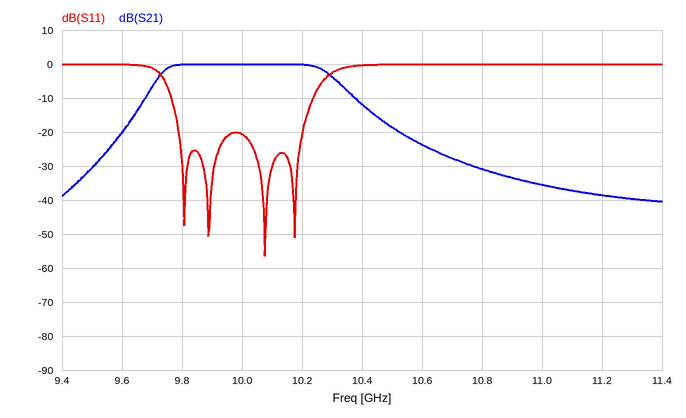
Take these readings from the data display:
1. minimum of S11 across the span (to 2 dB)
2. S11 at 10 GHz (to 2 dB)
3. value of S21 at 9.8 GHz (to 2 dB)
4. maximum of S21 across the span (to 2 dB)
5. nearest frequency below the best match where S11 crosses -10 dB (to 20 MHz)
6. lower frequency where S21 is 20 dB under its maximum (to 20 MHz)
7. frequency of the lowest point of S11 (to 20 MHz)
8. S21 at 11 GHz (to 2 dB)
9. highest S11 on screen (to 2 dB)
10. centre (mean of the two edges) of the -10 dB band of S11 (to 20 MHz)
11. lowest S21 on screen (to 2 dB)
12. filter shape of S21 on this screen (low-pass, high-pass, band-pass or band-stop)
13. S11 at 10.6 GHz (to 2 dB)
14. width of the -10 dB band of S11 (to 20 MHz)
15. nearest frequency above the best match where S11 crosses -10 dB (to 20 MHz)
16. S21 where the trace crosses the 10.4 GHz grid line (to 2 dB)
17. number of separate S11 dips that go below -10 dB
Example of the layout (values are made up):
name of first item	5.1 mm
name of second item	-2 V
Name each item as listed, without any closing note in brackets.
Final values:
minimum of S11 across the span	-56 dB
S11 at 10 GHz	-20 dB
value of S21 at 9.8 GHz	0 dB
maximum of S21 across the span	0 dB
nearest frequency below the best match where S11 crosses -10 dB	9.76 GHz
lower frequency where S21 is 20 dB under its maximum	9.60 GHz
frequency of the lowest point of S11	10.08 GHz
S21 at 11 GHz	-36 dB
highest S11 on screen	0 dB
centre (mean of the two edges) of the -10 dB band of S11	10.00 GHz
lowest S21 on screen	-40 dB
filter shape of S21 on this screen	band-pass
S11 at 10.6 GHz	0 dB
width of the -10 dB band of S11	480 MHz
nearest frequency above the best match where S11 crosses -10 dB	10.24 GHz
S21 where the trace crosses the 10.4 GHz grid line	-12 dB
number of separate S11 dips that go below -10 dB	4
